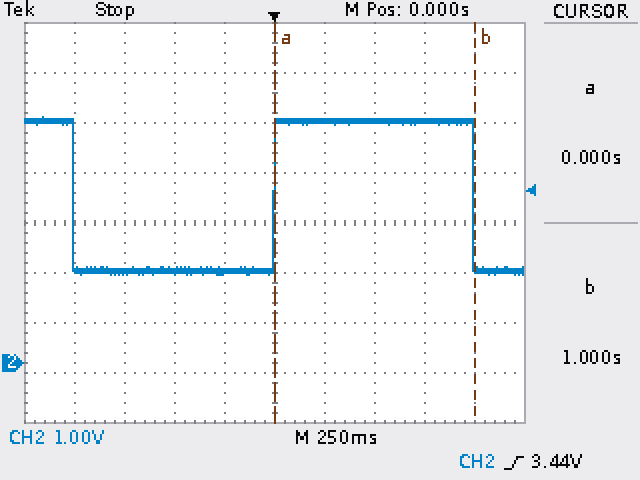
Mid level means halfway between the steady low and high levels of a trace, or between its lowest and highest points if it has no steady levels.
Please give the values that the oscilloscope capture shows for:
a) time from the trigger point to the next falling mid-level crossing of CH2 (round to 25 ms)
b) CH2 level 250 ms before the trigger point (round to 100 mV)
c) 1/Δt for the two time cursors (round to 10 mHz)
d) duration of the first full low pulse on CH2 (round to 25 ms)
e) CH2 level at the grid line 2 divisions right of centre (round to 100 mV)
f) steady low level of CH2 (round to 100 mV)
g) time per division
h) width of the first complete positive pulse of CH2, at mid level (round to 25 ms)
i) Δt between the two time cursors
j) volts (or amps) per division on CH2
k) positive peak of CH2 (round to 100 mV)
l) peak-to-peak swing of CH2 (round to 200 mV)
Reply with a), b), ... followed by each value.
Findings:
a) 1.000 s
b) 1.8 V
c) 1.00 Hz
d) 1.000 s
e) 4.8 V
f) 1.8 V
g) 250 ms
h) 1.000 s
i) 1.000 s
j) 1 V
k) 4.9 V
l) 3.2 V
